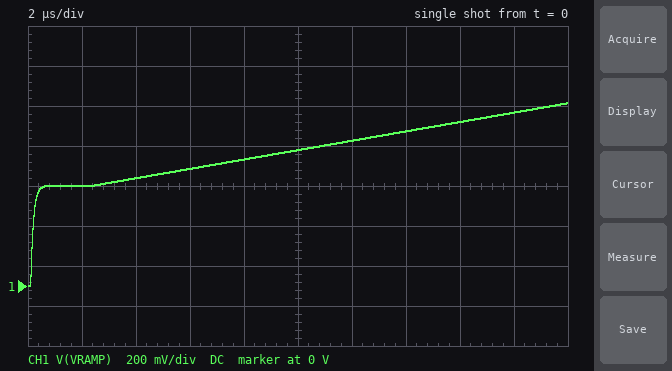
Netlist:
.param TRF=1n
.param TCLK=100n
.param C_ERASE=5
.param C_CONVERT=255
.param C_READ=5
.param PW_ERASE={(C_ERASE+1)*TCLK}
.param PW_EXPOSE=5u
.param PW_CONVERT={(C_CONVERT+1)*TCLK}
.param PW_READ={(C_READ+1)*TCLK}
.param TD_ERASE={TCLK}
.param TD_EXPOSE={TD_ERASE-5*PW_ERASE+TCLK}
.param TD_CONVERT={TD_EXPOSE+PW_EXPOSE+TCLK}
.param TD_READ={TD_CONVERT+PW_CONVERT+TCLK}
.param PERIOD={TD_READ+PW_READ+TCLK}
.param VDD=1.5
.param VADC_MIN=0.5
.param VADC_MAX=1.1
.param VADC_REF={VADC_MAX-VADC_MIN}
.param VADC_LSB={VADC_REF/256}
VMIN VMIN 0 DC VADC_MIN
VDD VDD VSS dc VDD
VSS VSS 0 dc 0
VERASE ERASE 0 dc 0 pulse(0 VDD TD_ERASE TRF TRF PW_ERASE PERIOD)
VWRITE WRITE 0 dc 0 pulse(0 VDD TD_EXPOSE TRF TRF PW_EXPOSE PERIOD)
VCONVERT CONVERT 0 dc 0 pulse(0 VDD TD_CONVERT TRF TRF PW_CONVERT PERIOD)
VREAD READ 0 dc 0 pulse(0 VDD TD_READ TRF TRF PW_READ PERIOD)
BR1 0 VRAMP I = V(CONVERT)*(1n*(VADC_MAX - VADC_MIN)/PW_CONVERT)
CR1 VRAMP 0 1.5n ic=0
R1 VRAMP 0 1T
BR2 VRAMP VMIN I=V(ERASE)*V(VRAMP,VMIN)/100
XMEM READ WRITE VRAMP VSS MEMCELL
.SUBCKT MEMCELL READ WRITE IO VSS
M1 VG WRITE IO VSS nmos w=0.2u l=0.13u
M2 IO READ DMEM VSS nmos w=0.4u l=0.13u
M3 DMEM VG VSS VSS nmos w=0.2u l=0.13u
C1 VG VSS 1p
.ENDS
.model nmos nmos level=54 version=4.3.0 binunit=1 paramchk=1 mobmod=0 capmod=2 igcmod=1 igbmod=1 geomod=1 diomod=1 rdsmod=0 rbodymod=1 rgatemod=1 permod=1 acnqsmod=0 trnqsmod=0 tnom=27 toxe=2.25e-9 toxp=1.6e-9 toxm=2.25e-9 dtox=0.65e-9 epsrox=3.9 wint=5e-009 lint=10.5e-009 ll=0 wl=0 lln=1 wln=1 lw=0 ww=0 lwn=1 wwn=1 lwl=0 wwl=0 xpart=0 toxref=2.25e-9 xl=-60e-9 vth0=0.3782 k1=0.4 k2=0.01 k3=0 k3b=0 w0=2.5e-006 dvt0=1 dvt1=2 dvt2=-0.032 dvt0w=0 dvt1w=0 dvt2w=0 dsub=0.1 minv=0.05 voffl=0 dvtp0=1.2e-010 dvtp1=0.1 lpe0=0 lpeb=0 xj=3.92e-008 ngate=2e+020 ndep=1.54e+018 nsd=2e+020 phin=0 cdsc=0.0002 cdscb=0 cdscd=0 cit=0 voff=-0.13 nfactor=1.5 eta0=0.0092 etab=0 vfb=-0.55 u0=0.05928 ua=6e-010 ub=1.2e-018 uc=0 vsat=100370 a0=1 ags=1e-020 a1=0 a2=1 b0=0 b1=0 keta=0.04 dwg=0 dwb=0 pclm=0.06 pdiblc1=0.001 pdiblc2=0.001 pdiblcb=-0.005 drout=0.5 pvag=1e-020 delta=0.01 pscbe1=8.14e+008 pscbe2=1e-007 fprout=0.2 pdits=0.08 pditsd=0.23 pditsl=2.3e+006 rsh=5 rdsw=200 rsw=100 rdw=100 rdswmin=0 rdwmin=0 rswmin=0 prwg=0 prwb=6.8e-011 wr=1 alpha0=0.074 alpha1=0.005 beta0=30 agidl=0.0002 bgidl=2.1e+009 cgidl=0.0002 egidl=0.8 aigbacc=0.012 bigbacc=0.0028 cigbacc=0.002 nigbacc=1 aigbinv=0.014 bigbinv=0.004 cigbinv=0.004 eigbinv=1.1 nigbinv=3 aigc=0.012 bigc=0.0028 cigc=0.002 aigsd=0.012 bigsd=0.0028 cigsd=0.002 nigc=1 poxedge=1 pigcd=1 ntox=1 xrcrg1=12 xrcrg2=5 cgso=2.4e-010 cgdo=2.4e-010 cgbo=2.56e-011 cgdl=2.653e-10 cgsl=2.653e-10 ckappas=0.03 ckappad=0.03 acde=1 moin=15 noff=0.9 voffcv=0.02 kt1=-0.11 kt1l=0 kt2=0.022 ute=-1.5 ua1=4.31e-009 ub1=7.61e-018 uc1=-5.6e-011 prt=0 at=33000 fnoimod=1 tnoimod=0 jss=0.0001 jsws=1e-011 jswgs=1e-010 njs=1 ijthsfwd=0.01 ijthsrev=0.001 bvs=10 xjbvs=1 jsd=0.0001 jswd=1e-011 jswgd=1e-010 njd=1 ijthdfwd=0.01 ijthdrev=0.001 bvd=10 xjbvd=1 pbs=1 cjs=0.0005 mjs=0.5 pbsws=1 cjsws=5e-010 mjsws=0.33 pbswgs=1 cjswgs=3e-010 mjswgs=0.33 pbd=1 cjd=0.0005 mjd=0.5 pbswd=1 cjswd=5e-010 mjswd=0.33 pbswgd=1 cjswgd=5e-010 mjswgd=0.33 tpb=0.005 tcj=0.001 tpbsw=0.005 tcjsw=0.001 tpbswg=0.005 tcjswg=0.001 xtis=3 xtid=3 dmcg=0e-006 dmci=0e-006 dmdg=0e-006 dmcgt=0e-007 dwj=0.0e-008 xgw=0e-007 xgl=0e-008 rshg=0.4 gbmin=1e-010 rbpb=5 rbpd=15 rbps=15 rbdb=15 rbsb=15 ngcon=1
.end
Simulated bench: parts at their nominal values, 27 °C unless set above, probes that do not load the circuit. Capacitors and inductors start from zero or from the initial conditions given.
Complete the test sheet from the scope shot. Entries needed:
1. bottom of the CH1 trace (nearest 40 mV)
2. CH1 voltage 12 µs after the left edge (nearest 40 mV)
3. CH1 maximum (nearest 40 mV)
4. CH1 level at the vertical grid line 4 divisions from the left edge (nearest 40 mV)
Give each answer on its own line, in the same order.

0 V
720 mV
920 mV
640 mV
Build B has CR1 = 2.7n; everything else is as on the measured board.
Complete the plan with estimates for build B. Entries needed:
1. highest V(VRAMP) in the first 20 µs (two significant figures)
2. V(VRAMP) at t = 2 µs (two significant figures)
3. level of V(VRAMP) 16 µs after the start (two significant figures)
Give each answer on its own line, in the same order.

710 mV
480 mV
660 mV
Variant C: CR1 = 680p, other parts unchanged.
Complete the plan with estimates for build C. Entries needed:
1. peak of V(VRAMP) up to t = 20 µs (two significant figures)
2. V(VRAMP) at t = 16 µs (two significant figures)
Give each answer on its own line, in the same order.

1.4 V
1.2 V
